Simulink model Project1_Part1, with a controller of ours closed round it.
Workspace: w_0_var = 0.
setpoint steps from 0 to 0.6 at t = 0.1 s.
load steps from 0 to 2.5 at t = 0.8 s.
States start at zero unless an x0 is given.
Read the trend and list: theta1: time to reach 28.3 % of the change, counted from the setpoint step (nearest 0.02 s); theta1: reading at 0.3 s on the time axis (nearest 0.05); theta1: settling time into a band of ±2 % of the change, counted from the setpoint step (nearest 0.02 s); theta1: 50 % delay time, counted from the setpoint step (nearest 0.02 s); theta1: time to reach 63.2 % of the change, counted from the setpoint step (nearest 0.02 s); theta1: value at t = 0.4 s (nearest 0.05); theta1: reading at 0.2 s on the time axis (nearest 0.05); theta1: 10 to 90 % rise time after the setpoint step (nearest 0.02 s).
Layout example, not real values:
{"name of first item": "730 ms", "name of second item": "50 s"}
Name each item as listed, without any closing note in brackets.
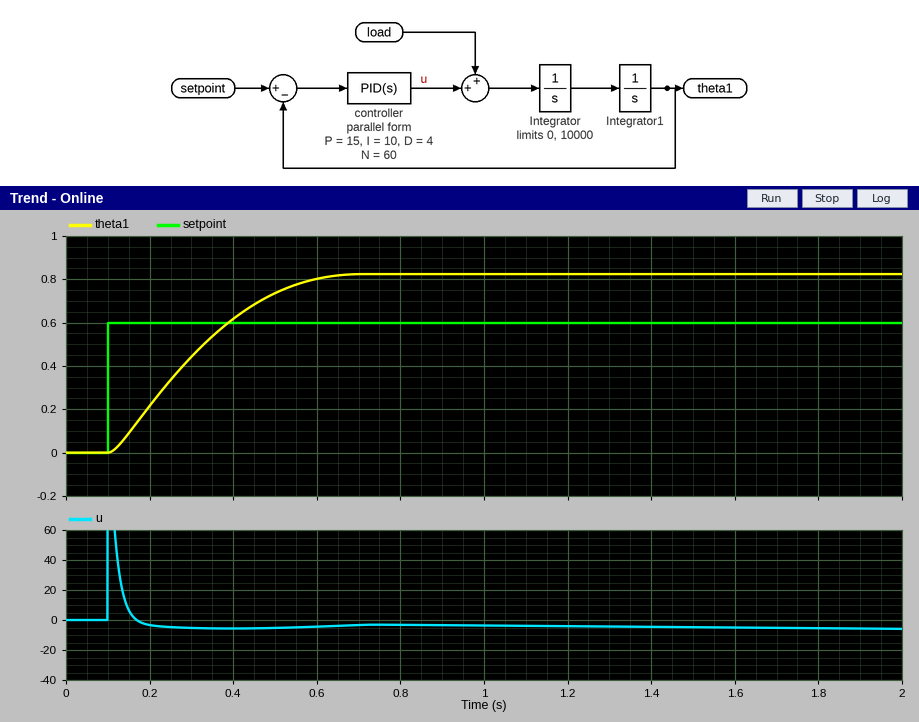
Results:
{"theta1: time to reach 28.3 % of the change, counted from the setpoint step": "0.10 s", "theta1: reading at 0.3 s on the time axis": "0.45", "theta1: settling time into a band of ±2 % of the change, counted from the setpoint step": "0.52 s", "theta1: 50 % delay time, counted from the setpoint step": "0.18 s", "theta1: time to reach 63.2 % of the change, counted from the setpoint step": "0.24 s", "theta1: value at t = 0.4 s": "0.60", "theta1: reading at 0.2 s on the time axis": "0.20", "theta1: 10 to 90 % rise time after the setpoint step": "0.36 s"}
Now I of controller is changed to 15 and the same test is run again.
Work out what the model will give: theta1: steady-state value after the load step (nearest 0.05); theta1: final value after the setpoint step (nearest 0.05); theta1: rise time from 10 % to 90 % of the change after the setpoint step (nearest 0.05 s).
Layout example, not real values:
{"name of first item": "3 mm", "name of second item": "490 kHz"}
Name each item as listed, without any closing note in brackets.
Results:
{"theta1: steady-state value after the load step": "0.85", "theta1: final value after the setpoint step": "0.85", "theta1: rise time from 10 % to 90 % of the change after the setpoint step": "0.35 s"}
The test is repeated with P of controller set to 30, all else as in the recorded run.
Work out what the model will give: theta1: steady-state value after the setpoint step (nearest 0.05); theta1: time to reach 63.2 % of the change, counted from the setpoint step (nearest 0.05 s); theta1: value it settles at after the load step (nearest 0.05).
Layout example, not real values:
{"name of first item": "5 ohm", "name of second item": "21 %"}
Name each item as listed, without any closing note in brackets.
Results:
{"theta1: steady-state value after the setpoint step": "0.85", "theta1: time to reach 63.2 % of the change, counted from the setpoint step": "0.20 s", "theta1: value it settles at after the load step": "0.85"}
